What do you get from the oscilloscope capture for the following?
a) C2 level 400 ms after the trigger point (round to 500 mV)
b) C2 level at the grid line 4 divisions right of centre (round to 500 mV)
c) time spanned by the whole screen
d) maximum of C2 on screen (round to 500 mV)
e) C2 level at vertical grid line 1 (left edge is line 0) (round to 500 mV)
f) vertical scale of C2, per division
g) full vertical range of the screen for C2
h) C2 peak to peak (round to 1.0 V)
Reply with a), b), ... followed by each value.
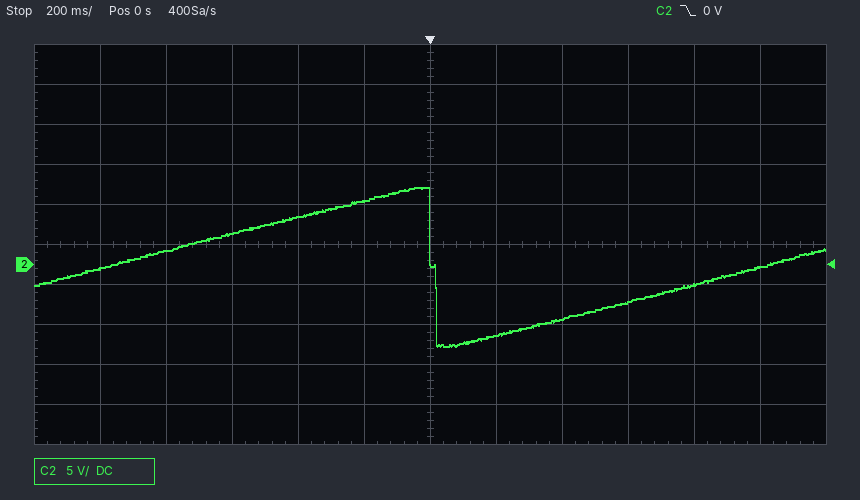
a) -7.0 V
b) -2.5 V
c) 2.4 s
d) 9.5 V
e) -500 mV
f) 5 V
g) 50 V
h) 20.0 V
